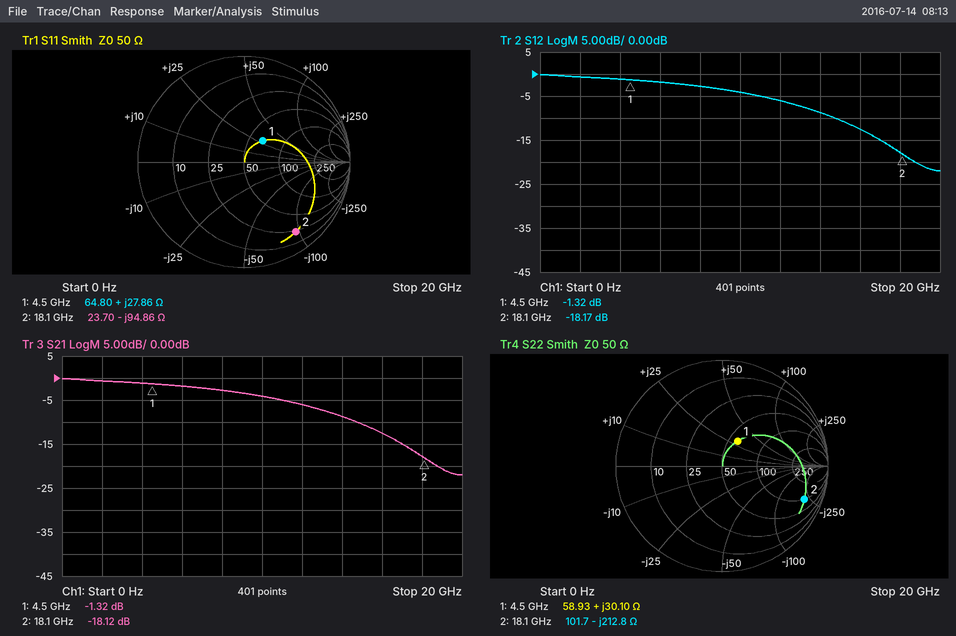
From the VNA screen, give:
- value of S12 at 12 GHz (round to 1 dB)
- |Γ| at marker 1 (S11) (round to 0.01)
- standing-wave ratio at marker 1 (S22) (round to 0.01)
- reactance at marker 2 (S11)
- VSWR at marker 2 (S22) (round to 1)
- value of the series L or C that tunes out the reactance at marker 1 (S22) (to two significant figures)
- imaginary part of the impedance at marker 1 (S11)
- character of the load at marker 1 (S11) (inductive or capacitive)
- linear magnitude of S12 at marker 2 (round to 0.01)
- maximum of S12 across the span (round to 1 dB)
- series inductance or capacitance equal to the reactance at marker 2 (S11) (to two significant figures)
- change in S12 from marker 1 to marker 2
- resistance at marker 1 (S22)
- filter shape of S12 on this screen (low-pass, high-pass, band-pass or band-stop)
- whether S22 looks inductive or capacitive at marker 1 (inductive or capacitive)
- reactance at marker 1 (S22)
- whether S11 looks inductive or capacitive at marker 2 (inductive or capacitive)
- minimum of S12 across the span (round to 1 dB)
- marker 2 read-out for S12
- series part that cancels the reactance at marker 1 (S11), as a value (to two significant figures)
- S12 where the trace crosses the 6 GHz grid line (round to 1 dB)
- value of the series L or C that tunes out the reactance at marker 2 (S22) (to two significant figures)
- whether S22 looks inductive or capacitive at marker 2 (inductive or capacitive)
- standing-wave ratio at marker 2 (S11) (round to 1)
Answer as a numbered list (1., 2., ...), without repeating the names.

1. -6 dB
2. 0.27
3. 1.77
4. -94.86 Ω
5. 11
6. 1.2 pF
7. +27.86 Ω
8. inductive
9. 0.12
10. 0 dB
11. 93 fF
12. -16.85 dB
13. 58.93 Ω
14. low-pass
15. inductive
16. +30.10 Ω
17. capacitive
18. -22 dB
19. -18.17 dB
20. 1.3 pF
21. -2 dB
22. 1.9 nH
23. capacitive
24. 10
